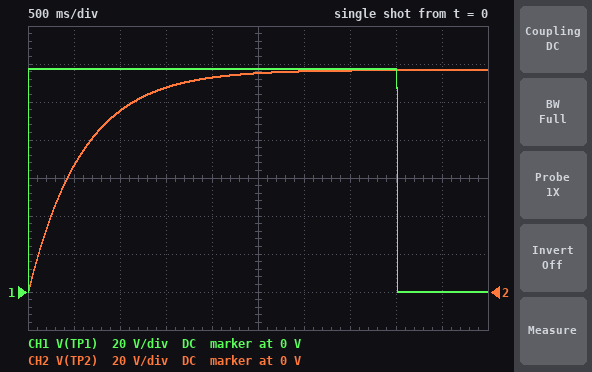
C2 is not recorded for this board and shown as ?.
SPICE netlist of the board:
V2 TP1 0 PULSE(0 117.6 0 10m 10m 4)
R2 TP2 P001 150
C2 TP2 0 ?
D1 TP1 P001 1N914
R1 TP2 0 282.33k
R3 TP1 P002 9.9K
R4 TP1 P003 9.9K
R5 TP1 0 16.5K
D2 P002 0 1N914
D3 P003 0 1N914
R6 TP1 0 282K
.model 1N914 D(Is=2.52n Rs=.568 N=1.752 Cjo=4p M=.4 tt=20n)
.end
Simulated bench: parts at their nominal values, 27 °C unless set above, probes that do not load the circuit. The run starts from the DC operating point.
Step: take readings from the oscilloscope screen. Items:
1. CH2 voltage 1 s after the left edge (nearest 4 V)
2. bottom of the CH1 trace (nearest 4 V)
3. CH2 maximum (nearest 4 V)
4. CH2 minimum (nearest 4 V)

96 V
0 V
116 V
0 V
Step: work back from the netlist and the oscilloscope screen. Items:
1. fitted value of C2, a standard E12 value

3.9 mF
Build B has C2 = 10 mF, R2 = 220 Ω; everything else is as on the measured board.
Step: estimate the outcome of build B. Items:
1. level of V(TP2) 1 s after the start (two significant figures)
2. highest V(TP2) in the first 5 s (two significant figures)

42 V
98 V
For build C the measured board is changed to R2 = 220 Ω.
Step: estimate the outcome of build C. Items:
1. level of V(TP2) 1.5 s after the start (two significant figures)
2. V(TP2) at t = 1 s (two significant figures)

96 V
80 V
